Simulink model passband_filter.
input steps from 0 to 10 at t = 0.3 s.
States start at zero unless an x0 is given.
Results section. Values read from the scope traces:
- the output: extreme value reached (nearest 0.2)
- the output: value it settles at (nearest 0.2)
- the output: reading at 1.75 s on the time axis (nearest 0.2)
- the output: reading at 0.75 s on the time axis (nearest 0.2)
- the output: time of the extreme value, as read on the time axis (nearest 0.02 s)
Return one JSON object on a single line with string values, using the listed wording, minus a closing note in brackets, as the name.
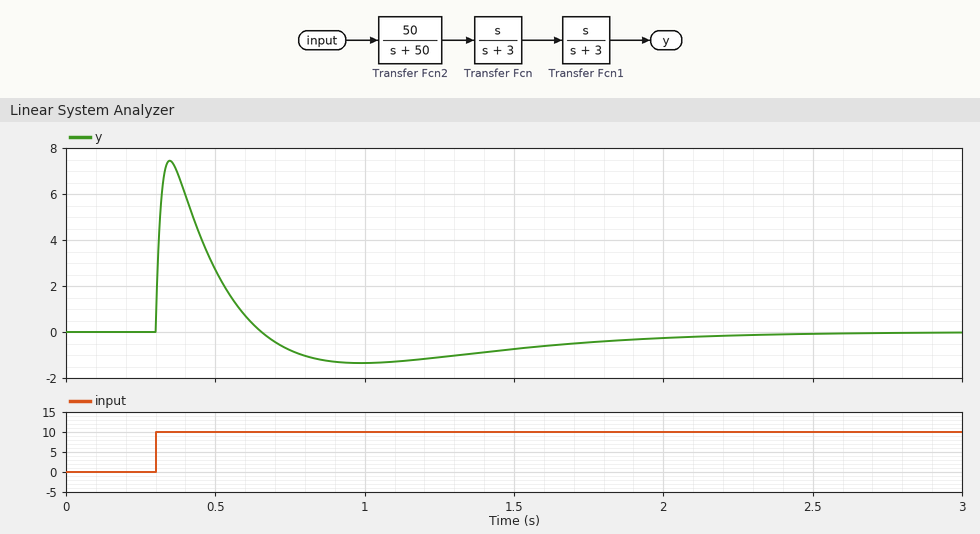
{"the output: extreme value reached": "7.4", "the output: value it settles at": "0.0", "the output: reading at 1.75 s on the time axis": "-0.4", "the output: reading at 0.75 s on the time axis": "-0.8", "the output: time of the extreme value, as read on the time axis": "0.34 s"}
